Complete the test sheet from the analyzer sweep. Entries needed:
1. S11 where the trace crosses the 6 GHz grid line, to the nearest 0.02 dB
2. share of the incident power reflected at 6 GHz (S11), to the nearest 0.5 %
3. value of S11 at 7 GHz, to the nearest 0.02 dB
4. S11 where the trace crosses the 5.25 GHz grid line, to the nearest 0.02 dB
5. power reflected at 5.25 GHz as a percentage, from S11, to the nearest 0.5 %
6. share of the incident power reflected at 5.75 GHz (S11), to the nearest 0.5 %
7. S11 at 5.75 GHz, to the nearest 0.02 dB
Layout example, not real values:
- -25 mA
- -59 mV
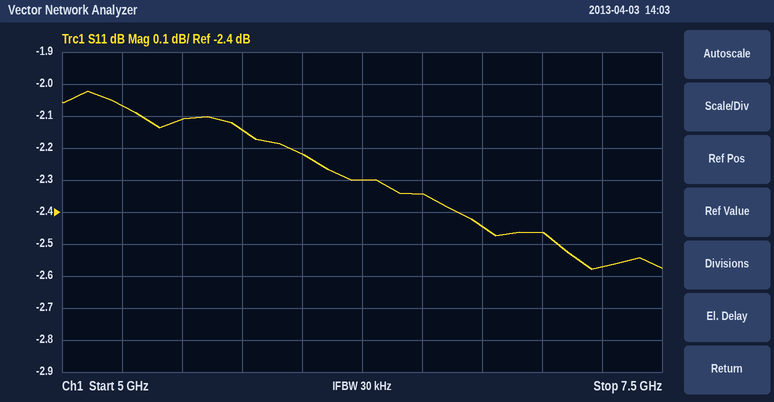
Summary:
- -2.22 dB
- 60.0 %
- -2.46 dB
- -2.06 dB
- 62.0 %
- 61.0 %
- -2.14 dB
